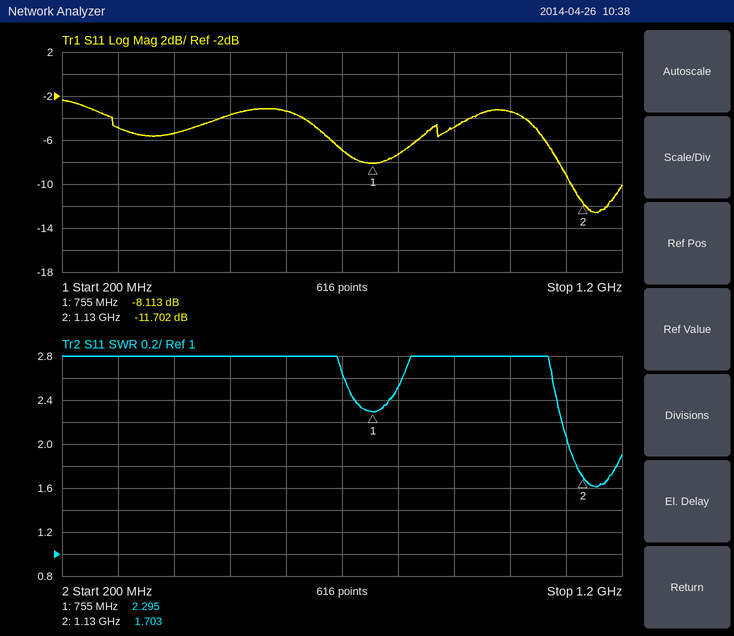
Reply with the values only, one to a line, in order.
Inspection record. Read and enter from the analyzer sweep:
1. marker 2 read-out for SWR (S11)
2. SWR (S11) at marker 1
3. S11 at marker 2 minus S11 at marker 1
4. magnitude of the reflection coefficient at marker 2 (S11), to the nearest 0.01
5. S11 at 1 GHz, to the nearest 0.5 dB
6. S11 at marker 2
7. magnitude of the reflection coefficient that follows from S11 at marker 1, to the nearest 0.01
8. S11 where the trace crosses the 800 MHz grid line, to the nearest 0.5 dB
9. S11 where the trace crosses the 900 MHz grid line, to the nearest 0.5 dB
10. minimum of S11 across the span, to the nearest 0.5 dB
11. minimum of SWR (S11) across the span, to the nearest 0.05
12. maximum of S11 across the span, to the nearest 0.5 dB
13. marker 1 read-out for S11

1.703
2.295
-3.589 dB
0.26
-3.5 dB
-11.702 dB
0.39
-7.5 dB
-5.0 dB
-12.5 dB
1.60
-2.5 dB
-8.113 dB
